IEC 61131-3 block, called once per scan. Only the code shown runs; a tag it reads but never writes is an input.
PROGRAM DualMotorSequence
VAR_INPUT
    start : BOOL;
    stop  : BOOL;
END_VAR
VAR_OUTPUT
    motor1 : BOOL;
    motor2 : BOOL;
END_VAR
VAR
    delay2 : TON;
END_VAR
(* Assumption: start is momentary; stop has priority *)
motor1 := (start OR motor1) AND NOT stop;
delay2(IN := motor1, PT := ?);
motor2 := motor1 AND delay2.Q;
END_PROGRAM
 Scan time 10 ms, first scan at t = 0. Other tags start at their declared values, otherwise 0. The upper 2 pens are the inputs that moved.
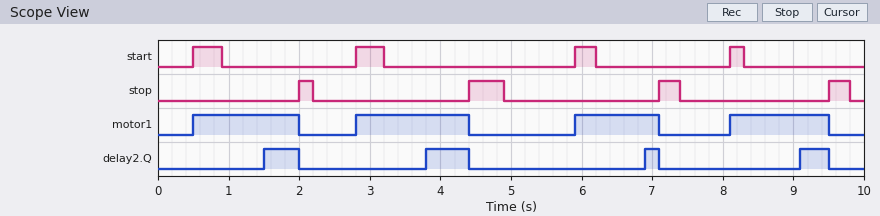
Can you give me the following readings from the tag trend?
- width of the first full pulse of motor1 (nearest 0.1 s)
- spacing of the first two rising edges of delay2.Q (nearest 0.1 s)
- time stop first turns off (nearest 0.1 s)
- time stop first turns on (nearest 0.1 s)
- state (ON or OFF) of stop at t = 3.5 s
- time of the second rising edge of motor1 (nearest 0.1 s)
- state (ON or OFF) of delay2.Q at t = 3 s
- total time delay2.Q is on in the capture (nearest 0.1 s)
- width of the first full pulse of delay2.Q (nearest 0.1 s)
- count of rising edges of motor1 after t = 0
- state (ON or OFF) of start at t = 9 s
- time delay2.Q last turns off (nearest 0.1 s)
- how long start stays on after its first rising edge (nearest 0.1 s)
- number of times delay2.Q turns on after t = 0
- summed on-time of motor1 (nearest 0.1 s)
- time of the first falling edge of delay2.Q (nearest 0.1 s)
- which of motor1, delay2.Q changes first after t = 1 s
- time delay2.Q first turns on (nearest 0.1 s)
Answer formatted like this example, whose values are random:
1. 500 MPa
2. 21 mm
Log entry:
1. 1.5 s
2. 2.3 s
3. 2.2 s
4. 2.0 s
5. OFF
6. 2.8 s
7. OFF
8. 1.7 s
9. 0.5 s
10. 4
11. OFF
12. 9.5 s
13. 0.4 s
14. 4
15. 5.7 s
16. 2.0 s
17. delay2.Q
18. 1.5 s
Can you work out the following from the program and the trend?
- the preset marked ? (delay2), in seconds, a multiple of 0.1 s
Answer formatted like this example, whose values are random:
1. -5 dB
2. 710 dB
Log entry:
1. 1.0 s
